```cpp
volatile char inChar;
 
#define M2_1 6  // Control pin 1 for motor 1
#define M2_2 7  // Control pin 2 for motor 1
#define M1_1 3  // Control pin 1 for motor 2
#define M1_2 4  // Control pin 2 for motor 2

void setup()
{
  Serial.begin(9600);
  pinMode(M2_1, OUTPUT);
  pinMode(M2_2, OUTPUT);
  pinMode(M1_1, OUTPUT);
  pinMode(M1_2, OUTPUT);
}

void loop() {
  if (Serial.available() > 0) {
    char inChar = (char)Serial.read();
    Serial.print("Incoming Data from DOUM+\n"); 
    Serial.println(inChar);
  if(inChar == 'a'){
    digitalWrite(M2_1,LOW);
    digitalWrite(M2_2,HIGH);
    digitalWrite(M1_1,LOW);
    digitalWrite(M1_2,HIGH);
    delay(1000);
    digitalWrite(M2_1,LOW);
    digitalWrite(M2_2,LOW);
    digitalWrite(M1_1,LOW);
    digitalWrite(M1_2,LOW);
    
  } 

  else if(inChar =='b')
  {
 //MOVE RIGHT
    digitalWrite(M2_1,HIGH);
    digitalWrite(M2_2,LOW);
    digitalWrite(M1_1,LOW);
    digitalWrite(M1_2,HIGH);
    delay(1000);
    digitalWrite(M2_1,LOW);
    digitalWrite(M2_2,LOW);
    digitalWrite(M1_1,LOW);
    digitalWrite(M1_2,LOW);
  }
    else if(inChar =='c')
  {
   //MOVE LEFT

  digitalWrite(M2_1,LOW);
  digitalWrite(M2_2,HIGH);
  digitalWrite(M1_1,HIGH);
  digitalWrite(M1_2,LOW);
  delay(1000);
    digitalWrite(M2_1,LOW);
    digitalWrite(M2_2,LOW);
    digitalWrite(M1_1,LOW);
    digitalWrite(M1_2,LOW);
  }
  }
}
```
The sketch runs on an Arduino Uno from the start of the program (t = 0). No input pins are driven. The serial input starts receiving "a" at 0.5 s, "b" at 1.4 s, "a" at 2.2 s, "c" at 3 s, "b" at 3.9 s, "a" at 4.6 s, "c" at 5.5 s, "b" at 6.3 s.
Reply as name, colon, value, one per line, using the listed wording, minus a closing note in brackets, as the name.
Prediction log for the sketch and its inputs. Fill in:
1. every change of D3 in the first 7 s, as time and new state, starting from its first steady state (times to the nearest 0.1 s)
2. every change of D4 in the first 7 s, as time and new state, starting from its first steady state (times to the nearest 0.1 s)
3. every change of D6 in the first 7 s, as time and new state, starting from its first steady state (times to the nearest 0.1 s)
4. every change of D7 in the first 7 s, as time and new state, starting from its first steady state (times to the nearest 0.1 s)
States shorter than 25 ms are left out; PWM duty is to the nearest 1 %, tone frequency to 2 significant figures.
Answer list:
every change of D3 in the first 7 s, as time and new state, starting from its first steady state: 0 s low; 3.5 s high; 4.5 s low; 6.5 s high
every change of D4 in the first 7 s, as time and new state, starting from its first steady state: 0 s low; 0.5 s high; 3.5 s low; 4.5 s high; 6.5 s low
every change of D6 in the first 7 s, as time and new state, starting from its first steady state: 0 s low; 1.5 s high; 2.5 s low; 4.5 s high; 5.5 s low
every change of D7 in the first 7 s, as time and new state, starting from its first steady state: 0 s low; 0.5 s high; 1.5 s low; 2.5 s high; 4.5 s low; 5.5 s high
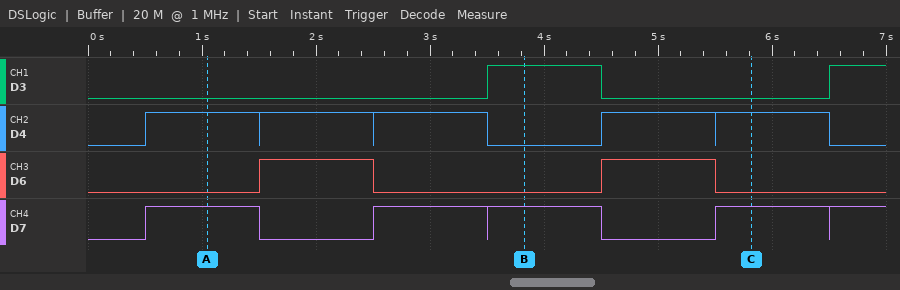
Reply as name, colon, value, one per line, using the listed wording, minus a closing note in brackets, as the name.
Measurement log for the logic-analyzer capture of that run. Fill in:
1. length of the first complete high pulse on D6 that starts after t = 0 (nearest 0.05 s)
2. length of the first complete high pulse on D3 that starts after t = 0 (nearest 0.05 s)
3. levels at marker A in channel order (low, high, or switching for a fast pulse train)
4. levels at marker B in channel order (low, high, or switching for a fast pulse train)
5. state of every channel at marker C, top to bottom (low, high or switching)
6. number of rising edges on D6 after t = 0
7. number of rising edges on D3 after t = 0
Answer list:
length of the first complete high pulse on D6 that starts after t = 0: 1.00 s
length of the first complete high pulse on D3 that starts after t = 0: 1.00 s
levels at marker A in channel order: D3 low, D4 high, D6 low, D7 high
levels at marker B in channel order: D3 high, D4 low, D6 low, D7 high
state of every channel at marker C, top to bottom: D3 low, D4 high, D6 low, D7 high
number of rising edges on D6 after t = 0: 2
number of rising edges on D3 after t = 0: 2
